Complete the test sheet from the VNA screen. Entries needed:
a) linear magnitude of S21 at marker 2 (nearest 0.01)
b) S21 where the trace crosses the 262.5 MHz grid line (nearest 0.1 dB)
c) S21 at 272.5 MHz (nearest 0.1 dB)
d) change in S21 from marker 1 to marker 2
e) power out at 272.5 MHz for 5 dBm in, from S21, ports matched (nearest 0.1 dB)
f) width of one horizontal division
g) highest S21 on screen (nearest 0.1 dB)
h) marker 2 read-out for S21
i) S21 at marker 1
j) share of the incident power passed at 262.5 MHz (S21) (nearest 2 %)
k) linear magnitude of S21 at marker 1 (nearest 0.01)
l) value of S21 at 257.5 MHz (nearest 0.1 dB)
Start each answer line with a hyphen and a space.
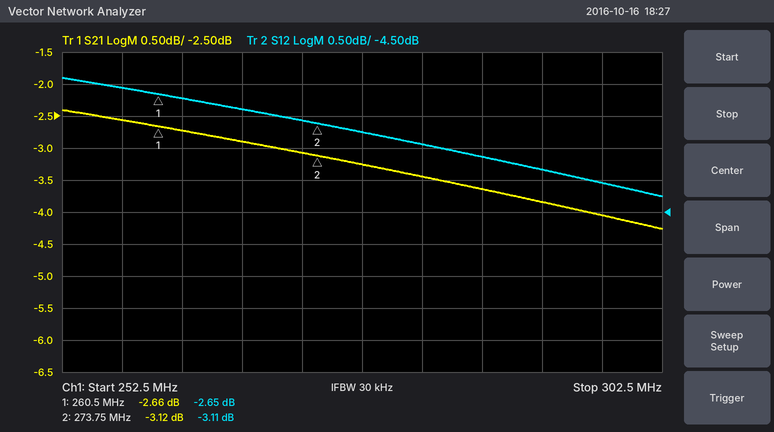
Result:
- 0.70
- -2.7 dB
- -3.1 dB
- -0.46 dB
- 1.9 dBm
- 5 MHz
- -2.4 dB
- -3.12 dB
- -2.66 dB
- 54 %
- 0.74
- -2.6 dB
